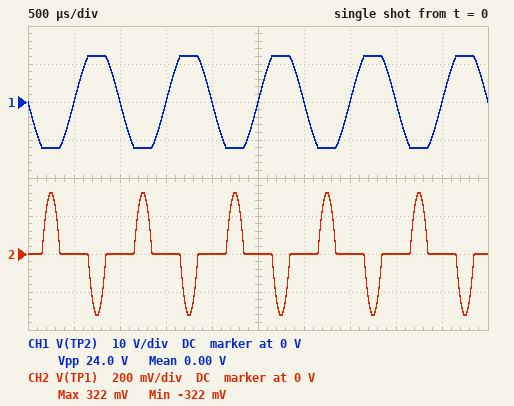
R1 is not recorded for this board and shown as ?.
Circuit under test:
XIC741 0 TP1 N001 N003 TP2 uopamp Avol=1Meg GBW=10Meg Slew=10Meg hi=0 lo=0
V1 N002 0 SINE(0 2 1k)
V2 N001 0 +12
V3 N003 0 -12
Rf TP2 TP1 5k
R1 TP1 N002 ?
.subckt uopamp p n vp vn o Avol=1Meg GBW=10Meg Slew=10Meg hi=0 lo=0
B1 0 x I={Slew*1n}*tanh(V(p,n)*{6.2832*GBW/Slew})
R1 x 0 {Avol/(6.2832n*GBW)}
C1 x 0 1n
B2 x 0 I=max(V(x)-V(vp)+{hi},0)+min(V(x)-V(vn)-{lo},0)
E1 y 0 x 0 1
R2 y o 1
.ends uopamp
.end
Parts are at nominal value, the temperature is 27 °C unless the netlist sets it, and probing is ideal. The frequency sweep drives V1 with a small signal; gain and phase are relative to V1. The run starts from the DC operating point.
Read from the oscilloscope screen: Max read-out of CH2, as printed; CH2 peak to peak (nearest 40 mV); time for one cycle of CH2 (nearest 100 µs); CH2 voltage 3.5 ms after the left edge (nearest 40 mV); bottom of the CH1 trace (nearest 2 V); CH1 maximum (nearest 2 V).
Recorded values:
322 mV
640 mV
1.0 ms
0 V
-12 V
12 V
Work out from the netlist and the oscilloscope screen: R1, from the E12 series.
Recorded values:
680 Ω
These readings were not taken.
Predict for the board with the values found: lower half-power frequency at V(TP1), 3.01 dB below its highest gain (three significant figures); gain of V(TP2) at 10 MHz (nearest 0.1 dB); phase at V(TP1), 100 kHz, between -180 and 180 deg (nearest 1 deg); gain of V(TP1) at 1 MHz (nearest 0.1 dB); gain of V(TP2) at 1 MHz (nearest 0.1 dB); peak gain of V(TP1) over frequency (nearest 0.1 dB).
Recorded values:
1.20 MHz
-1.2 dB
85 deg
-5.0 dB
15.0 dB
-1.1 dB
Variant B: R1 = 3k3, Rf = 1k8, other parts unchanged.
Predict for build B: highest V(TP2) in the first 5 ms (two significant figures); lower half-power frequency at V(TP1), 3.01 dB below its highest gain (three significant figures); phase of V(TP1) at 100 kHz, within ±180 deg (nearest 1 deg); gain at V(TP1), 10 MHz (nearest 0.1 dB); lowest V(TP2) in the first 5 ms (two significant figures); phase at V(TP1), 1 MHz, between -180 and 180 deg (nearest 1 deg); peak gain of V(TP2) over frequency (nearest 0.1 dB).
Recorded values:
1.1 V
6.47 MHz
89 deg
-10.6 dB
-1.1 V
81 deg
-5.3 dB
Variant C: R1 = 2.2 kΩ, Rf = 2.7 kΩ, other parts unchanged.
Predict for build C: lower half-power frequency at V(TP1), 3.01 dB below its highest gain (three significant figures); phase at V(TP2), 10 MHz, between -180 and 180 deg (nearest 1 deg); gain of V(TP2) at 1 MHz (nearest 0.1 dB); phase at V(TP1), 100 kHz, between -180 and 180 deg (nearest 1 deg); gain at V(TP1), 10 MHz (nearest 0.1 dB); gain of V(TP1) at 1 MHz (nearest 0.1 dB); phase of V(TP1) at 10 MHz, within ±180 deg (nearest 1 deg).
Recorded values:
4.49 MHz
114 deg
1.6 dB
89 deg
-6.0 dB
-18.4 dB
24 deg
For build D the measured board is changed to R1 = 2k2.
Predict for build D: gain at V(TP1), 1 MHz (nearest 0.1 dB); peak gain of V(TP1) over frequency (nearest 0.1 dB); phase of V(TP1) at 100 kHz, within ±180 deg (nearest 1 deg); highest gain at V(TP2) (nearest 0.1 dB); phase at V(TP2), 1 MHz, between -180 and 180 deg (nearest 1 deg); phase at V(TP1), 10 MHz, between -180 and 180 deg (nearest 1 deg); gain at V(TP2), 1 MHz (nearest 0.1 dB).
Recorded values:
-13.3 dB
-3.2 dB
88 deg
7.1 dB
162 deg
17 deg
6.7 dB
